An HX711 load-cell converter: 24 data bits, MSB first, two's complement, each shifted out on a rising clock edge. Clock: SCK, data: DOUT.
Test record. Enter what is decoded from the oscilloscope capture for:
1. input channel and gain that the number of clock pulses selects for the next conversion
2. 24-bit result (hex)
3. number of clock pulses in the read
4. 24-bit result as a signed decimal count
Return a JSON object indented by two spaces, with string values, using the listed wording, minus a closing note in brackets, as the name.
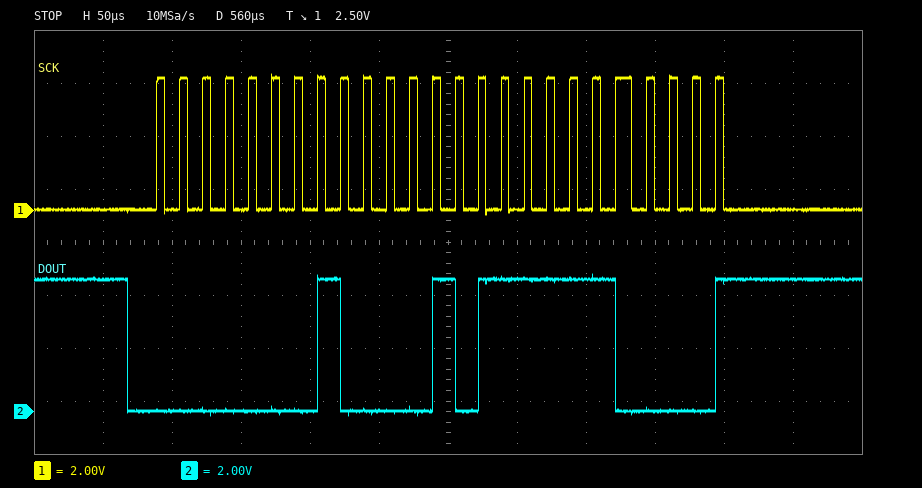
{
  "input channel and gain that the number of clock pulses selects for the next conversion": "channel A, gain 128",
  "24-bit result": "0x010BF0",
  "number of clock pulses in the read": "25",
  "24-bit result as a signed decimal count": "68592"
}
